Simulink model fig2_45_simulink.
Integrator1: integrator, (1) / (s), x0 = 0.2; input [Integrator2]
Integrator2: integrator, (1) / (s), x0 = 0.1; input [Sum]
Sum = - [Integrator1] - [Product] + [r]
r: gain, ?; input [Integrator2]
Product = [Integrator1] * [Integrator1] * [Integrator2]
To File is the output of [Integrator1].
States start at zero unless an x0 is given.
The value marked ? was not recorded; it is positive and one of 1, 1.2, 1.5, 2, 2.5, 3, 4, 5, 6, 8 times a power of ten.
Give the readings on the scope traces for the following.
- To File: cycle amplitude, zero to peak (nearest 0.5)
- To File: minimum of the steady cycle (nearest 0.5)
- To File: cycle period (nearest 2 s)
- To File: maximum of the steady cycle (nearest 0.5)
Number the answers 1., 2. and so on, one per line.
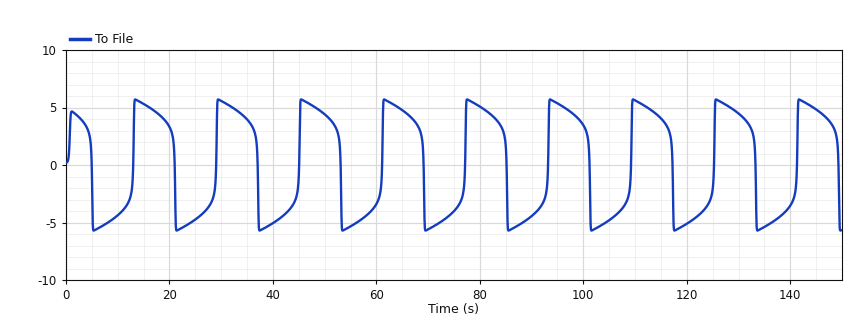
1. 5.5
2. -5.5
3. 16 s
4. 5.5
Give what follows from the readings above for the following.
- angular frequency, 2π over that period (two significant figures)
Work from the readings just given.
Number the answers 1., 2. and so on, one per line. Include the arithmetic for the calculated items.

1. 2π / 16 = 0.39 rad/s
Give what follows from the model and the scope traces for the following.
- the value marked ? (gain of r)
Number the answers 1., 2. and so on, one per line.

1. 8
